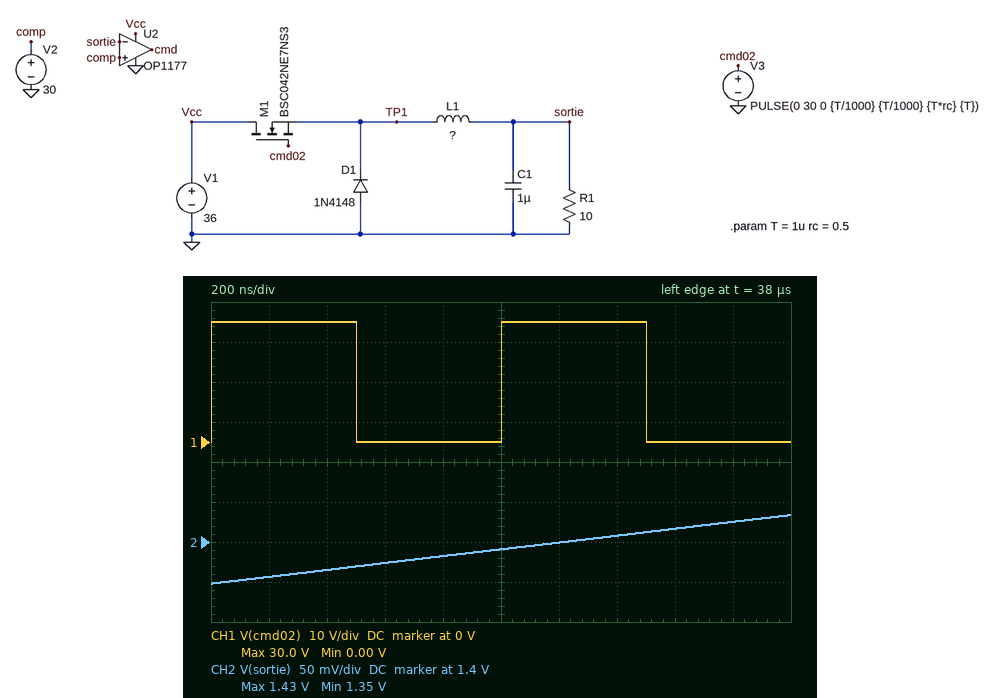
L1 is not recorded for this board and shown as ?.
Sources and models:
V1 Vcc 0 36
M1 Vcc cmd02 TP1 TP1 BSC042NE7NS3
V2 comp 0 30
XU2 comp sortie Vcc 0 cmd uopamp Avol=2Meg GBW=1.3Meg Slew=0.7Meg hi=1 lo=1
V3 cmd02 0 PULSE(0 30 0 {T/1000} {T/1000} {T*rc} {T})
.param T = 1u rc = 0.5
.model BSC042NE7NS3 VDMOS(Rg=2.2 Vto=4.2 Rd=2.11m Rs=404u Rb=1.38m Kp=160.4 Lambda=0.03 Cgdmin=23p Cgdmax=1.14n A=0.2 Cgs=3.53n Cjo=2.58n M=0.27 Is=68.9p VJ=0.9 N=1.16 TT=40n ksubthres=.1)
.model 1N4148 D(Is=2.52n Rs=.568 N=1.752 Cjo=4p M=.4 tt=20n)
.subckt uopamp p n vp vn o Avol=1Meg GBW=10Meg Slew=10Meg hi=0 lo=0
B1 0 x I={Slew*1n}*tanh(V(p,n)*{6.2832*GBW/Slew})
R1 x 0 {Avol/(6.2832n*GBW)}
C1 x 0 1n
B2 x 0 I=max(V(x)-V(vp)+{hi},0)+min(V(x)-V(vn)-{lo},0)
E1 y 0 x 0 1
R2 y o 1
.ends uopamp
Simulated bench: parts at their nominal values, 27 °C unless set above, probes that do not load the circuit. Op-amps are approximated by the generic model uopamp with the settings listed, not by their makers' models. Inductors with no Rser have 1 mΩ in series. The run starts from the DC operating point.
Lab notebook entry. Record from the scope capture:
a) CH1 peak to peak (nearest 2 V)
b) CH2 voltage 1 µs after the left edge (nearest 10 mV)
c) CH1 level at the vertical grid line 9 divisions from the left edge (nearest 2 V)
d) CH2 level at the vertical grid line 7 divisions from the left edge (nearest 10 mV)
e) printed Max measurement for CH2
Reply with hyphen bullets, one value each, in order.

- 30 V
- 1.39 V
- 0 V
- 1.41 V
- 1.43 V
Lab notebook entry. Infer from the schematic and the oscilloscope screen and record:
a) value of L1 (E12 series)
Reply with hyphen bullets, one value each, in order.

- 2.7 mH
